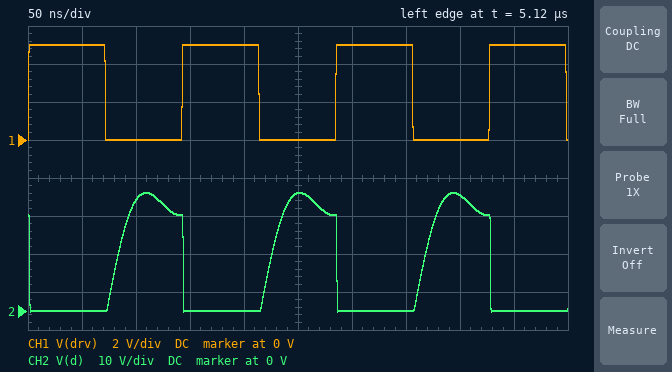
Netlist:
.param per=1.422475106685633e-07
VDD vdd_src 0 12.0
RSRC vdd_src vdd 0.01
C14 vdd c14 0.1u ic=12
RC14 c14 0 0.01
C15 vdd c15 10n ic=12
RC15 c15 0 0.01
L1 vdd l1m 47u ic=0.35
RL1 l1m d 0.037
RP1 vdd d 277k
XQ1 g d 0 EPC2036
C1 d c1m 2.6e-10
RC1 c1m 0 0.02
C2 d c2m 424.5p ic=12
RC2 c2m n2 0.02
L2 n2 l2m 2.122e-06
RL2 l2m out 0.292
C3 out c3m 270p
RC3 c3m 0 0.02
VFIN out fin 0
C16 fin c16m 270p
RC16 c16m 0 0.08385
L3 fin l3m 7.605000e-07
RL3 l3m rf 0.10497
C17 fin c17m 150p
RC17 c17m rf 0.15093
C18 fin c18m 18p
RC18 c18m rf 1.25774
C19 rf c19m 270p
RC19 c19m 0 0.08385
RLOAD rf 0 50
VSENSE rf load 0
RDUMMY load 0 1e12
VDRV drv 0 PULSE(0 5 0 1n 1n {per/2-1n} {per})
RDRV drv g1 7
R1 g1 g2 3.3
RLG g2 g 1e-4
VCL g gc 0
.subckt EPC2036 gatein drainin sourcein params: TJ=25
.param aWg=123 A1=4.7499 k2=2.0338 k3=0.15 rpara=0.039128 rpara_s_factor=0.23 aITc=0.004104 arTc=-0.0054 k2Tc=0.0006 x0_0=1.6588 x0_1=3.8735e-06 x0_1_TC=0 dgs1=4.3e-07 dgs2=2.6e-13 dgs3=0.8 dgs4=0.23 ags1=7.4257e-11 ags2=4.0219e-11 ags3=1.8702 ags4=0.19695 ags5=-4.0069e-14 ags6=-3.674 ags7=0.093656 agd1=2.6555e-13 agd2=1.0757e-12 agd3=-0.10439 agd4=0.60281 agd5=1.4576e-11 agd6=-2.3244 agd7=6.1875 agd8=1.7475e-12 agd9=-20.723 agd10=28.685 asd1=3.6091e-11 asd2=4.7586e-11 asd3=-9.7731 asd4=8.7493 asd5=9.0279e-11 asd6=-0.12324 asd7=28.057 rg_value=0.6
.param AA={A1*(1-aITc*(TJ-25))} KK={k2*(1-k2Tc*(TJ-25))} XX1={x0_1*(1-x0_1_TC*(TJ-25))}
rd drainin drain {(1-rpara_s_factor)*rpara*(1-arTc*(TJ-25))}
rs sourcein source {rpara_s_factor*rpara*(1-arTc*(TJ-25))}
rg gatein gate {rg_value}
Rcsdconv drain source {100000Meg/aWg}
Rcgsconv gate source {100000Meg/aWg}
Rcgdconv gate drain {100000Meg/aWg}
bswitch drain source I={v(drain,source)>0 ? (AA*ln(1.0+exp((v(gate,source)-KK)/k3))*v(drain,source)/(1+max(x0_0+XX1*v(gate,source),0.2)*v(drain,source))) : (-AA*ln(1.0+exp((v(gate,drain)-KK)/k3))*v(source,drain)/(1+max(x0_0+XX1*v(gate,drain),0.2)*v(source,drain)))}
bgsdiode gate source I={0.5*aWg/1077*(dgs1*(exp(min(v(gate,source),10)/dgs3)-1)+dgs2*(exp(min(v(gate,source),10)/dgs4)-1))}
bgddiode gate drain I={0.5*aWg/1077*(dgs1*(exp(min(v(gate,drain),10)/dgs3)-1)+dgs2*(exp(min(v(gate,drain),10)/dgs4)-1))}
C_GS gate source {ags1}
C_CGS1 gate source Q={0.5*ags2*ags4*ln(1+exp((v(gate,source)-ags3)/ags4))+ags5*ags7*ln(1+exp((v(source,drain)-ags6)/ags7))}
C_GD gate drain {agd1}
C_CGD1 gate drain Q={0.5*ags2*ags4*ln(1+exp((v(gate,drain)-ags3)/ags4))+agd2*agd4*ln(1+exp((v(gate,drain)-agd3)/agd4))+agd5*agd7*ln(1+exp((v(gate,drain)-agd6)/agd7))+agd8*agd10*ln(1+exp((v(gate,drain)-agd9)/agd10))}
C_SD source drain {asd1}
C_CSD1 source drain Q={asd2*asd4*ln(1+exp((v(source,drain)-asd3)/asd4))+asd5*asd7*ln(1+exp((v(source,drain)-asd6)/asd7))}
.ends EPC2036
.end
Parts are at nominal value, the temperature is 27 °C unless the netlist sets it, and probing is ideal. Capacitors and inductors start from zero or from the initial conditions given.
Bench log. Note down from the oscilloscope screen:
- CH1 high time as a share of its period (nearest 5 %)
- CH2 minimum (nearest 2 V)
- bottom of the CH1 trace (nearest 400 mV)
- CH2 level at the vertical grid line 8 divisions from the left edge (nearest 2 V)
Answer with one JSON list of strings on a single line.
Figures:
["50 %", "0 V", "0 V", "30 V"]
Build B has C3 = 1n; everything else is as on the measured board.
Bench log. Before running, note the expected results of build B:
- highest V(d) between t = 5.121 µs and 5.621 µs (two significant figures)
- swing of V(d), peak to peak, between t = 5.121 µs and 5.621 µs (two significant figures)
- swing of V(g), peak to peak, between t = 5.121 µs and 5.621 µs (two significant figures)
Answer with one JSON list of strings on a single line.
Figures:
["47 V", "49 V", "5.2 V"]
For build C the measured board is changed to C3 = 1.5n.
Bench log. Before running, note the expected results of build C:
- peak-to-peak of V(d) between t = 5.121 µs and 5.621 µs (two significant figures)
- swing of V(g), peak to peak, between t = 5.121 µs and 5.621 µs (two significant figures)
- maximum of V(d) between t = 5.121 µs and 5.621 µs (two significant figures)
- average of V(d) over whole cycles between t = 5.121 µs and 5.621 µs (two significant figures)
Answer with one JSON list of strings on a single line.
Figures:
["50 V", "5.2 V", "48 V", "13 V"]
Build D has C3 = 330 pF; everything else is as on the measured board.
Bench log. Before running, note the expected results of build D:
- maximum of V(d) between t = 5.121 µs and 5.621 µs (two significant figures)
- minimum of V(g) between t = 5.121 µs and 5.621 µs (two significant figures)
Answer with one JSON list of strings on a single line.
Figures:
["32 V", "-5.0 mV"]
